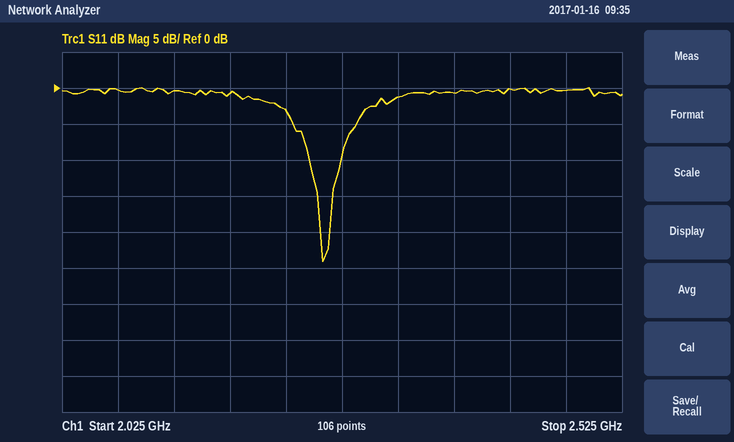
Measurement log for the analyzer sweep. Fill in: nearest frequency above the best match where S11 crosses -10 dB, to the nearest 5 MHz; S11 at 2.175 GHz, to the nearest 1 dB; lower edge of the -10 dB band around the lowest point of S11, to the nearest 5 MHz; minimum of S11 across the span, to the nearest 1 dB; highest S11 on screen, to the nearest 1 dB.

2.275 GHz
-1 dB
2.245 GHz
-24 dB
0 dB
